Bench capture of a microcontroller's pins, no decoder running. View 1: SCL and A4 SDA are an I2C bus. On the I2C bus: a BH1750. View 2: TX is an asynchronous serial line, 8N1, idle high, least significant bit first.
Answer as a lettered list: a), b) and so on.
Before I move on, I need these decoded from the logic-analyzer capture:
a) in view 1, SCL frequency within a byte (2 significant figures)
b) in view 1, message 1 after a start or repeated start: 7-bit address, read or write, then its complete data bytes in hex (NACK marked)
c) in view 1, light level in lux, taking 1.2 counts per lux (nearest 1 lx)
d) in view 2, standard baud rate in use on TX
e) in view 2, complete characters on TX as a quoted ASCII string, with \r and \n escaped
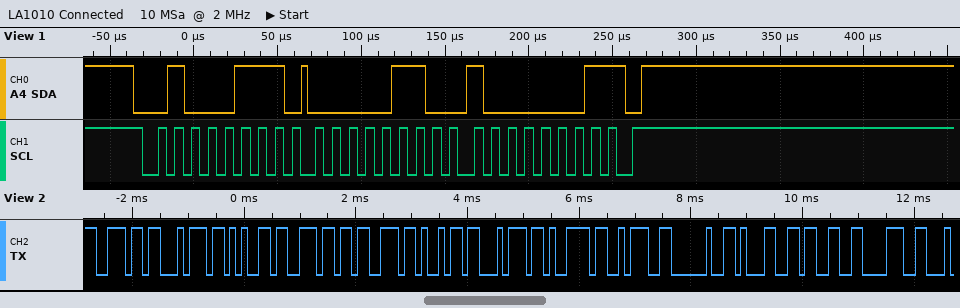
a) 100 kHz
b) 0x23 read: 06 81 NACK
c) 1388 lx
d) 9600 baud
e) "ntensity: 138"
